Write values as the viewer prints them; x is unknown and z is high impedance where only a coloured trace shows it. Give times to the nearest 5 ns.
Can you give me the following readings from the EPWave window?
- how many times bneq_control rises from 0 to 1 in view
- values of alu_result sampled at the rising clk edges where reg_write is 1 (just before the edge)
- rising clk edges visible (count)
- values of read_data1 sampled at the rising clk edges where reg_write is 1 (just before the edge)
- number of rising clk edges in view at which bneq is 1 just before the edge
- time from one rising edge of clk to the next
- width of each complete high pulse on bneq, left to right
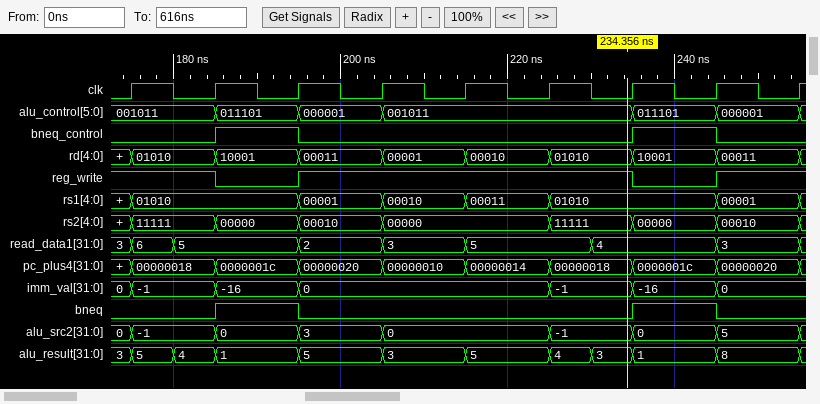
2
3, 4, 5, 3, 5, 3, 8
9
3, 5, 2, 3, 5, 4, 3
2
10 ns
10 ns, 10 ns
